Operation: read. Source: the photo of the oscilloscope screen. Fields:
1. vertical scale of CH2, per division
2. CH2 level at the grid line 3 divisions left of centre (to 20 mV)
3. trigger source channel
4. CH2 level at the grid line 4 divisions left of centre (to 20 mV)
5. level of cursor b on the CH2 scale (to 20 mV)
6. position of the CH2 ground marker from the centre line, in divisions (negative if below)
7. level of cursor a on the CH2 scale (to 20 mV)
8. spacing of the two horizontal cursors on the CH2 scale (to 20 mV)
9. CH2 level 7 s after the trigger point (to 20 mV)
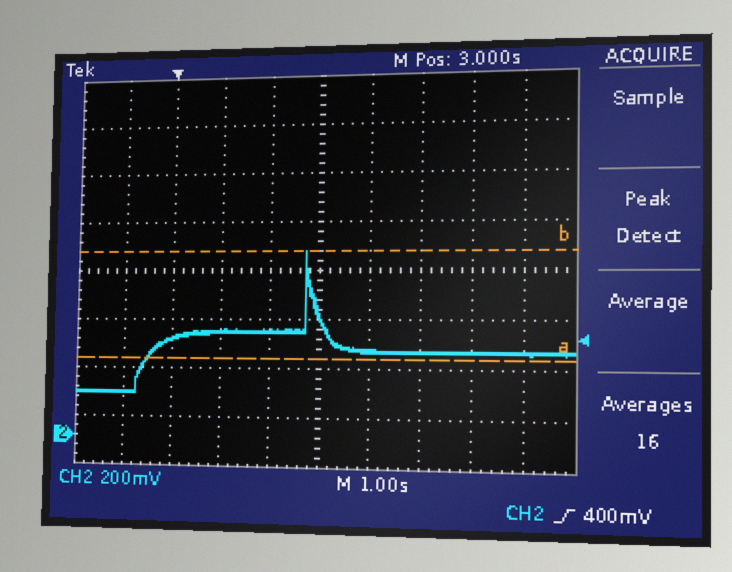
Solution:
200 mV
400 mV
CH2
180 mV
760 mV
-3.4 div
320 mV
440 mV
340 mV
